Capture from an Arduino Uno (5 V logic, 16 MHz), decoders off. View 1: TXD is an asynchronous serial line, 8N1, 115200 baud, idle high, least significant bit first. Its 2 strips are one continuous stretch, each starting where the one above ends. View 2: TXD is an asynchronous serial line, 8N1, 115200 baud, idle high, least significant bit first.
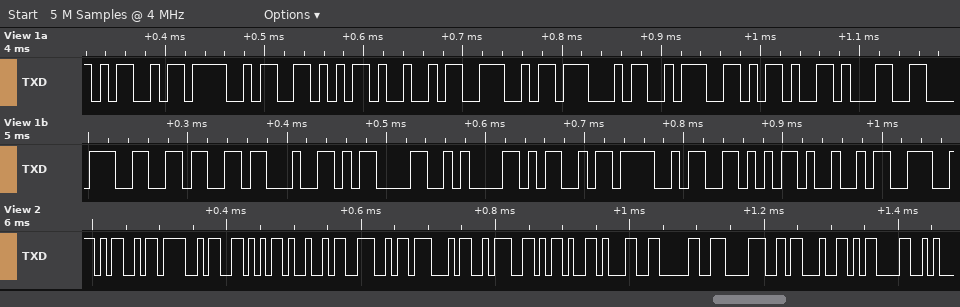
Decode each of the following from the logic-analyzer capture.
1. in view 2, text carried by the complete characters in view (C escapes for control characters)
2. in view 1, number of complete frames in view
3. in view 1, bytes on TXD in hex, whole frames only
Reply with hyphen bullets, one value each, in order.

- "MOVING:-108#\r"
- 18
- 4D 4F 56 49 4E 47 3A 2D 31 38 36 23 0D 0A 4D 4F 56 49
